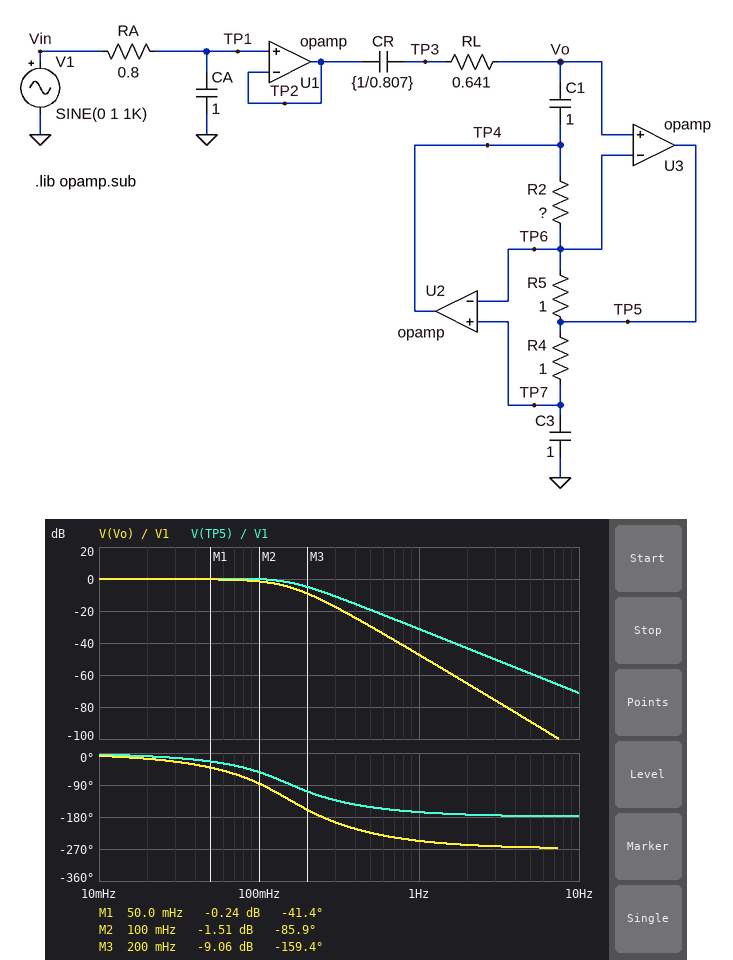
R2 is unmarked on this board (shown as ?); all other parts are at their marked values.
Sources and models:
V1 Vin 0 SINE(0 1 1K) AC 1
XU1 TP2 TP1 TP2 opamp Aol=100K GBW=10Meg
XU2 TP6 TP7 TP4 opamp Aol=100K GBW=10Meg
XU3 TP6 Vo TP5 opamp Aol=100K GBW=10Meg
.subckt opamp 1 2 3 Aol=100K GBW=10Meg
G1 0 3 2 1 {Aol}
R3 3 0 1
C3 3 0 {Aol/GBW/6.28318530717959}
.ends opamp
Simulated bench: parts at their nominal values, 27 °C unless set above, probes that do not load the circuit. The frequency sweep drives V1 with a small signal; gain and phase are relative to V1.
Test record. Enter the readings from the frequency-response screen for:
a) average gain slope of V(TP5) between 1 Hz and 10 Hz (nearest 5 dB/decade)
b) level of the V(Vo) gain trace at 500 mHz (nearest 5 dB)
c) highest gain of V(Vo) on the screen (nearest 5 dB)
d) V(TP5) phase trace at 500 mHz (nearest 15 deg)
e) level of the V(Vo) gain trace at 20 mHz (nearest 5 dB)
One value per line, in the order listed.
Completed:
-40 dB/decade
-30 dB
0 dB
-150 deg
0 dB
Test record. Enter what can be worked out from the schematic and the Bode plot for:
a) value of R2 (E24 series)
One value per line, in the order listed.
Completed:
1.8 Ω
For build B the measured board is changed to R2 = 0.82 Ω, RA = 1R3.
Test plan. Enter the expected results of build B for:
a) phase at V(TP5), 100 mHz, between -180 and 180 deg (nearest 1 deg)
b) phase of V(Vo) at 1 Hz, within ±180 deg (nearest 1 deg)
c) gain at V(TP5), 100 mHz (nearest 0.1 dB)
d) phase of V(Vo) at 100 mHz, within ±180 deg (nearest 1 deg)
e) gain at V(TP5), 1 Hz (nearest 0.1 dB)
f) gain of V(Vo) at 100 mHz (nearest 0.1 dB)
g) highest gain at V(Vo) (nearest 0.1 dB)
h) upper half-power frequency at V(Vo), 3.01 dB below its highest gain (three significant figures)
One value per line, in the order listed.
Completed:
-35 deg
109 deg
0.2 dB
-67 deg
-28.3 dB
-1.3 dB
0 dB
174 mHz
